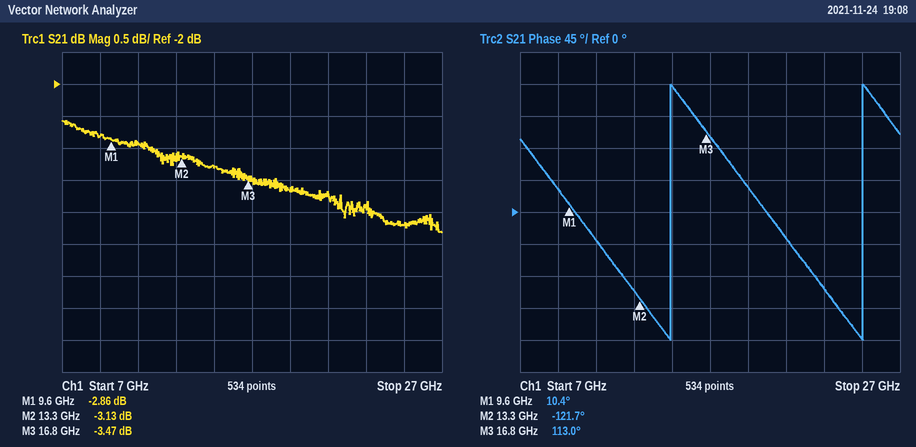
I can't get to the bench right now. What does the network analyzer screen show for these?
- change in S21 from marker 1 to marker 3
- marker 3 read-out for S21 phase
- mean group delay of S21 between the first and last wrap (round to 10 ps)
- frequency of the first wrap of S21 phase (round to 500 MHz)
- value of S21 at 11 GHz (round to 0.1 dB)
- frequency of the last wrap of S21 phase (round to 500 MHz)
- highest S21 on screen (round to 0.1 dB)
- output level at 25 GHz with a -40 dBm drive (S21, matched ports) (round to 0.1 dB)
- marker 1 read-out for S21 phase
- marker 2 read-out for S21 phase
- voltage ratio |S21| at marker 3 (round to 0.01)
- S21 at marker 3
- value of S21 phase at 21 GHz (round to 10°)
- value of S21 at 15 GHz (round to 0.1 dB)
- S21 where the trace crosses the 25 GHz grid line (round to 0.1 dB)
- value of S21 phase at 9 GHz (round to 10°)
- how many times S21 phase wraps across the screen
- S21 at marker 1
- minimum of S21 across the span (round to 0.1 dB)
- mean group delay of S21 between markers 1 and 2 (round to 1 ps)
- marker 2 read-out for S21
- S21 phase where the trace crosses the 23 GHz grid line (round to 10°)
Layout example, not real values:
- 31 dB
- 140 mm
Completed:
- -0.61 dB
- 113.0°
- 100 ps
- 15.0 GHz
- -2.9 dB
- 25.0 GHz
- -2.6 dB
- -44.2 dBm
- 10.4°
- -121.7°
- 0.67
- -3.47 dB
- -40°
- -3.3 dB
- -4.2 dB
- 30°
- 2
- -2.86 dB
- -4.3 dB
- 99 ps
- -3.13 dB
- -110°
